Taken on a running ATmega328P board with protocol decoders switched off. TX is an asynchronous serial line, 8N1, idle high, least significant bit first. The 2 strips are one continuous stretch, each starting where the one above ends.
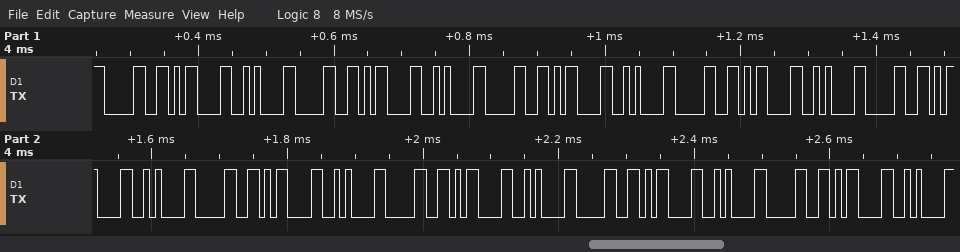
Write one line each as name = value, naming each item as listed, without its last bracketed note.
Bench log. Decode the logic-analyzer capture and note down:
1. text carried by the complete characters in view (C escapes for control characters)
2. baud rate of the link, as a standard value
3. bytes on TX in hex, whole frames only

text carried by the complete characters in view = "0\r\n0\r\n0\r\n0\r\n0\r\n0\r\n0\r\n0\r\n0\r\n"
baud rate of the link, as a standard value = 115200 baud
bytes on TX in hex, whole frames only = 30 0D 0A 30 0D 0A 30 0D 0A 30 0D 0A 30 0D 0A 30 0D 0A 30 0D 0A 30 0D 0A 30 0D 0A
